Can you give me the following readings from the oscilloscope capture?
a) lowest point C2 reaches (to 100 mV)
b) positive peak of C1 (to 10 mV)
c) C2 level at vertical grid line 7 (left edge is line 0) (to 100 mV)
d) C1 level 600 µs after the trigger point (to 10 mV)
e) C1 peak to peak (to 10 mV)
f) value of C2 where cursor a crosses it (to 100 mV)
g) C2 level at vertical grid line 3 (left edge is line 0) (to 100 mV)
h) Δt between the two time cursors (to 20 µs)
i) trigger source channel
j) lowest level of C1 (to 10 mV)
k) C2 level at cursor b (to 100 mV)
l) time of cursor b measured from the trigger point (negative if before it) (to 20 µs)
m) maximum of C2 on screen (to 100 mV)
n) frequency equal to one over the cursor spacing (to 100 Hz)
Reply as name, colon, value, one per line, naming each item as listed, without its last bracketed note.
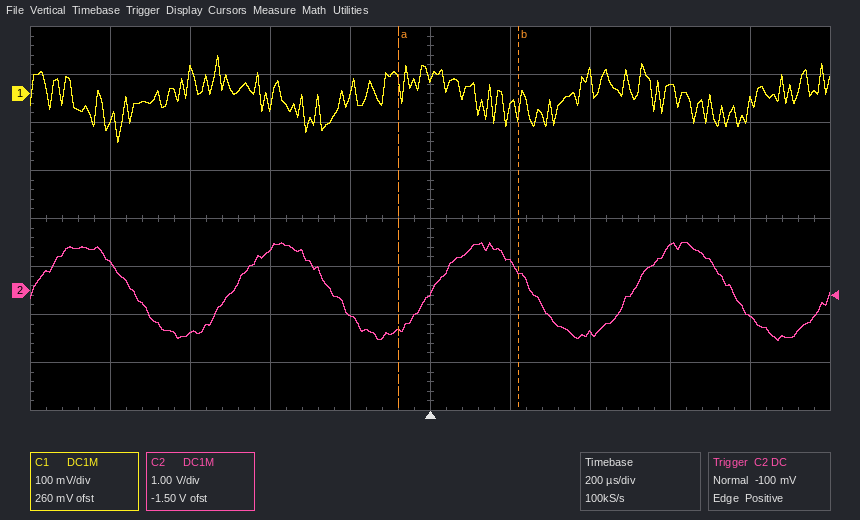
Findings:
lowest point C2 reaches: -1.0 V
positive peak of C1: 80 mV
C2 level at vertical grid line 7 (left edge is line 0): -900 mV
C1 level 600 µs after the trigger point: 20 mV
C1 peak to peak: 180 mV
value of C2 where cursor a crosses it: -800 mV
C2 level at vertical grid line 3 (left edge is line 0): 900 mV
Δt between the two time cursors: 300 µs
trigger source channel: C2
lowest level of C1: -100 mV
C2 level at cursor b: 400 mV
time of cursor b measured from the trigger point (negative if before it): +220 µs
maximum of C2 on screen: 1.0 V
frequency equal to one over the cursor spacing: 3.3 kHz
